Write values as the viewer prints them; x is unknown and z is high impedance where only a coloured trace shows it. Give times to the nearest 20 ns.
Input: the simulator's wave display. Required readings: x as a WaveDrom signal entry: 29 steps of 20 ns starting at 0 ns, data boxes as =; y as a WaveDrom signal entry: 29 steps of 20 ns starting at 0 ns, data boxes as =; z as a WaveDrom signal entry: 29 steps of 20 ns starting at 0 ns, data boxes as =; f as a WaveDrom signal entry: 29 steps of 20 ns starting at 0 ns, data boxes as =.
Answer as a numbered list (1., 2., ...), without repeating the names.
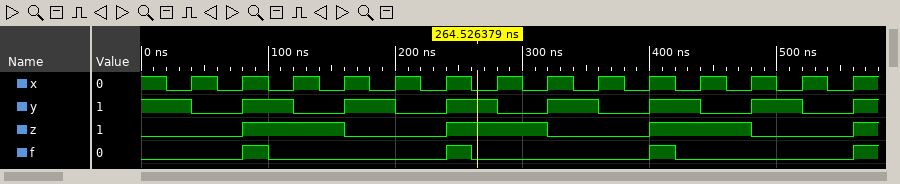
1. {name: 'x', wave: '10101010101010101010101010101'}
2. {name: 'y', wave: '1.0.1.0.1.0.1.0.1.0.1.0.1.0.1'}
3. {name: 'z', wave: '0...1...0...1...0...1...0...1'}
4. {name: 'f', wave: '0...10......10......10......1'}
